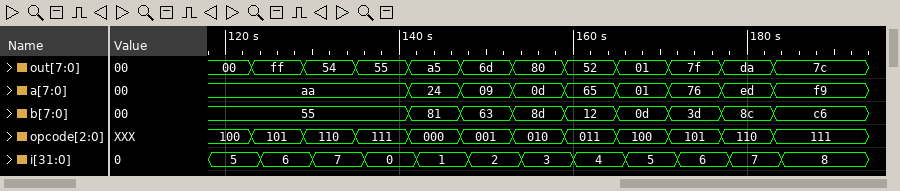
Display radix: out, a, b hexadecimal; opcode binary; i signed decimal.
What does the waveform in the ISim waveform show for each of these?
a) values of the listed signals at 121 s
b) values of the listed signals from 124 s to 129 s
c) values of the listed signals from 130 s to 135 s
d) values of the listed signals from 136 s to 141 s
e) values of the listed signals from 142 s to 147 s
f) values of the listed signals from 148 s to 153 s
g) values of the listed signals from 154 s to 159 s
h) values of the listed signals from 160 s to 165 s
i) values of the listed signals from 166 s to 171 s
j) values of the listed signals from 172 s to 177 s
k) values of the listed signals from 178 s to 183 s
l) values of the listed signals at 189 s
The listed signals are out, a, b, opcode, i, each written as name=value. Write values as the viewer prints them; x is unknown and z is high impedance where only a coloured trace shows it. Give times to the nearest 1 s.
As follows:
out=00, a=aa, b=55, opcode=100, i=5
out=ff, a=aa, b=55, opcode=101, i=6
out=54, a=aa, b=55, opcode=110, i=7
out=55, a=aa, b=55, opcode=111, i=0
out=a5, a=24, b=81, opcode=000, i=1
out=6d, a=09, b=63, opcode=001, i=2
out=80, a=0d, b=8d, opcode=010, i=3
out=52, a=65, b=12, opcode=011, i=4
out=01, a=01, b=0d, opcode=100, i=5
out=7f, a=76, b=3d, opcode=101, i=6
out=da, a=ed, b=8c, opcode=110, i=7
out=7c, a=f9, b=c6, opcode=111, i=8
